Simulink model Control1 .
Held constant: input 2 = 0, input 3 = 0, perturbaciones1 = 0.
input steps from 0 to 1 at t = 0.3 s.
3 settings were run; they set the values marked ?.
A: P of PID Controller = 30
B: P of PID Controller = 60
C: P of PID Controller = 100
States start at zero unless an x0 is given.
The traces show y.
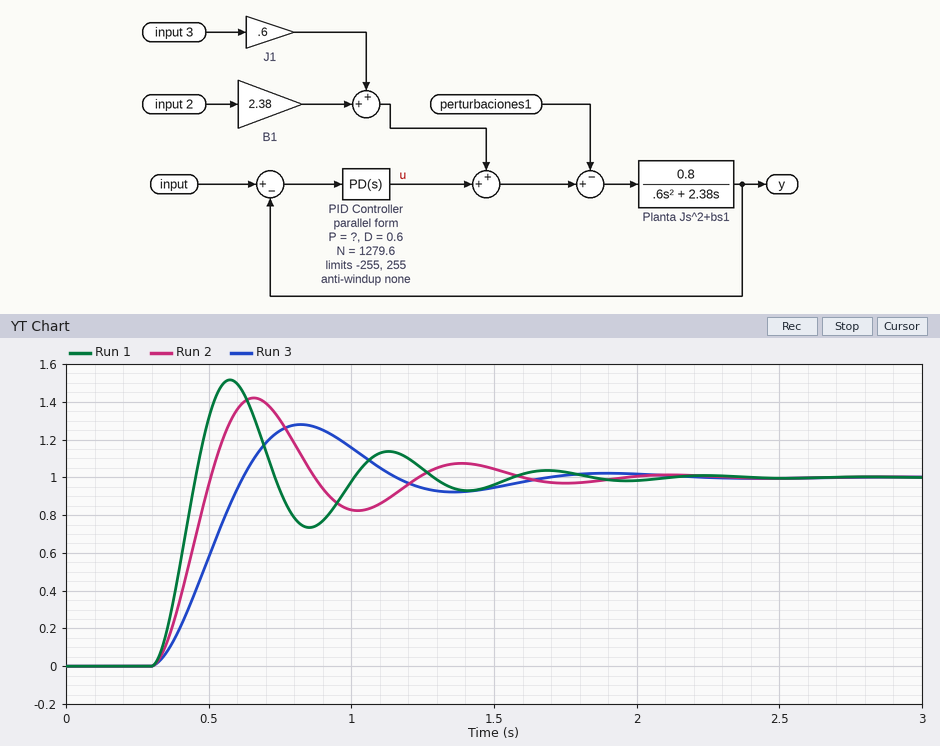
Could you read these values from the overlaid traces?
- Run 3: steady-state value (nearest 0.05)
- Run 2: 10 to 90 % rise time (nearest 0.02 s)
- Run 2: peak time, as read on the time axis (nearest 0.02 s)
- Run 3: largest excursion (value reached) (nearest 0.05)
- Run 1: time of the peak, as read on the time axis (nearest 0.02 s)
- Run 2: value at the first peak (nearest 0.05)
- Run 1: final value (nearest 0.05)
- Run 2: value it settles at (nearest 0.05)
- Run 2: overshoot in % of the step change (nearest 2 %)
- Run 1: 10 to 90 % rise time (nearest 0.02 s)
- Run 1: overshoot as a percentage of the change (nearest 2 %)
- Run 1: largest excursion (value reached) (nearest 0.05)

1.00
0.14 s
0.66 s
1.30
0.58 s
1.40
1.00
1.00
42 %
0.10 s
52 %
1.50
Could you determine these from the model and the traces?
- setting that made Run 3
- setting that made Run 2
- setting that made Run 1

A
B
C
